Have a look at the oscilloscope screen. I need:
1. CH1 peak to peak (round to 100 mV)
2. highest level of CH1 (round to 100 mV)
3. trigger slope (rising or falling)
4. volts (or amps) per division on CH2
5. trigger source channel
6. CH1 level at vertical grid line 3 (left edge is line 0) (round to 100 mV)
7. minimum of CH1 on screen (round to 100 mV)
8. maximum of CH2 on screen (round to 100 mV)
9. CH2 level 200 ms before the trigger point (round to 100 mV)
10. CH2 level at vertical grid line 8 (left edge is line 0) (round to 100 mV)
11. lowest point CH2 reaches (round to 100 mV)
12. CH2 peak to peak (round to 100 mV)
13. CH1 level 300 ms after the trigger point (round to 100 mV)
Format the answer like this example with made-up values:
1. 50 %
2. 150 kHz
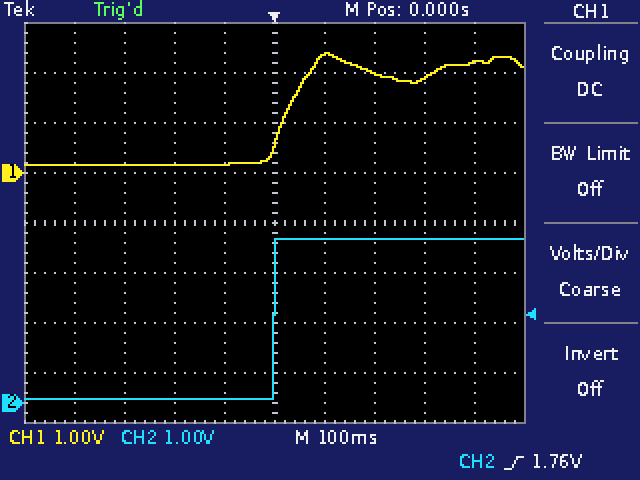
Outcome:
1. 2.2 V
2. 2.4 V
3. rising
4. 1 V
5. CH2
6. 200 mV
7. 200 mV
8. 3.3 V
9. 100 mV
10. 3.3 V
11. 100 mV
12. 3.2 V
13. 1.9 V
